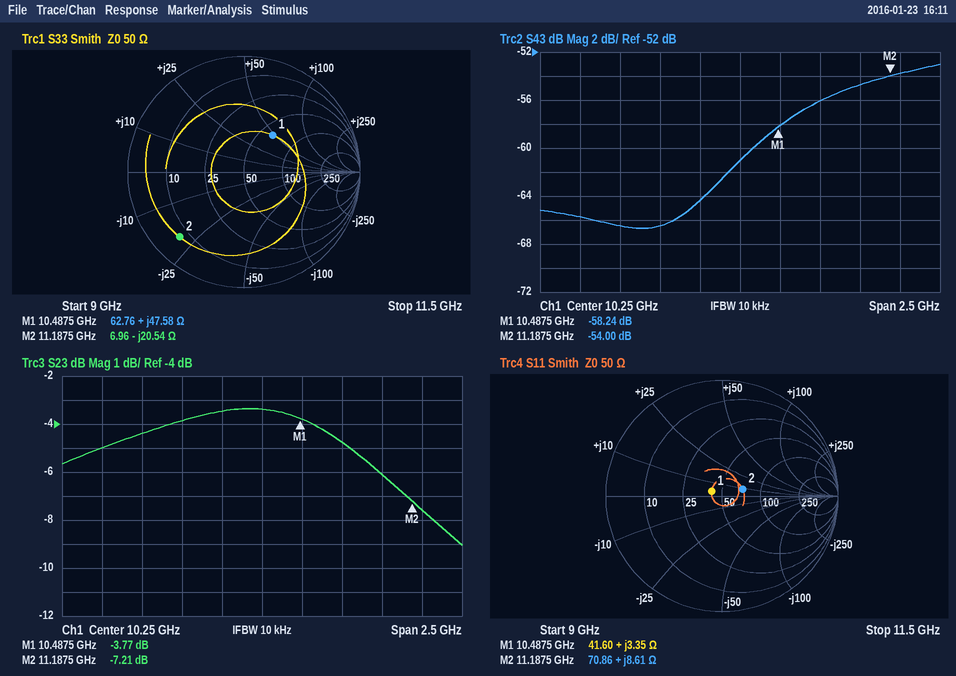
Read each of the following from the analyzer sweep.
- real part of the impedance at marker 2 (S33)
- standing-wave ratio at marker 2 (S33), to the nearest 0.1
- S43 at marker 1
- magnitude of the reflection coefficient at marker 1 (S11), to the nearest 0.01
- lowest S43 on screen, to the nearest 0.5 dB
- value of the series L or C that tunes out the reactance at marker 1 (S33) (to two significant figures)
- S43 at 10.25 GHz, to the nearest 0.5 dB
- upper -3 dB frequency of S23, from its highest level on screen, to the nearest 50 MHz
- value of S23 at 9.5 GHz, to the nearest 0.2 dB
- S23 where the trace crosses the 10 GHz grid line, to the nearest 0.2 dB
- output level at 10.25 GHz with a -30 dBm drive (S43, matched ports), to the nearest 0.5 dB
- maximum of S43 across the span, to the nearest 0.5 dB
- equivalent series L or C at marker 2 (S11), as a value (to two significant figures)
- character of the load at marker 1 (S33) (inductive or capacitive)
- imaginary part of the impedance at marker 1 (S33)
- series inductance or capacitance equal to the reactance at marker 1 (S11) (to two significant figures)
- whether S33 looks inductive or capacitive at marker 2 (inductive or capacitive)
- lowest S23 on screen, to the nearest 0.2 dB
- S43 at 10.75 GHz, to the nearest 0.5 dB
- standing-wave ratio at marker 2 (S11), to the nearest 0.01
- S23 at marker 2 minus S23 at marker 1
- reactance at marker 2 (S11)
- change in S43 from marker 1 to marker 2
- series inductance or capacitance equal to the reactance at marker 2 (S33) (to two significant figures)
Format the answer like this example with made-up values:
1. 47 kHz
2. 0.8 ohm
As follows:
1. 6.96 Ω
2. 8.4
3. -58.24 dB
4. 0.10
5. -66.5 dB
6. 320 fF
7. -61.0 dB
8. 11.05 GHz
9. -4.4 dB
10. -3.4 dB
11. -91.0 dBm
12. -53.0 dB
13. 120 pH
14. inductive
15. +47.58 Ω
16. 51 pH
17. capacitive
18. -9.0 dB
19. -56.0 dB
20. 1.46
21. -3.44 dB
22. +8.61 Ω
23. 4.24 dB
24. 690 fF
